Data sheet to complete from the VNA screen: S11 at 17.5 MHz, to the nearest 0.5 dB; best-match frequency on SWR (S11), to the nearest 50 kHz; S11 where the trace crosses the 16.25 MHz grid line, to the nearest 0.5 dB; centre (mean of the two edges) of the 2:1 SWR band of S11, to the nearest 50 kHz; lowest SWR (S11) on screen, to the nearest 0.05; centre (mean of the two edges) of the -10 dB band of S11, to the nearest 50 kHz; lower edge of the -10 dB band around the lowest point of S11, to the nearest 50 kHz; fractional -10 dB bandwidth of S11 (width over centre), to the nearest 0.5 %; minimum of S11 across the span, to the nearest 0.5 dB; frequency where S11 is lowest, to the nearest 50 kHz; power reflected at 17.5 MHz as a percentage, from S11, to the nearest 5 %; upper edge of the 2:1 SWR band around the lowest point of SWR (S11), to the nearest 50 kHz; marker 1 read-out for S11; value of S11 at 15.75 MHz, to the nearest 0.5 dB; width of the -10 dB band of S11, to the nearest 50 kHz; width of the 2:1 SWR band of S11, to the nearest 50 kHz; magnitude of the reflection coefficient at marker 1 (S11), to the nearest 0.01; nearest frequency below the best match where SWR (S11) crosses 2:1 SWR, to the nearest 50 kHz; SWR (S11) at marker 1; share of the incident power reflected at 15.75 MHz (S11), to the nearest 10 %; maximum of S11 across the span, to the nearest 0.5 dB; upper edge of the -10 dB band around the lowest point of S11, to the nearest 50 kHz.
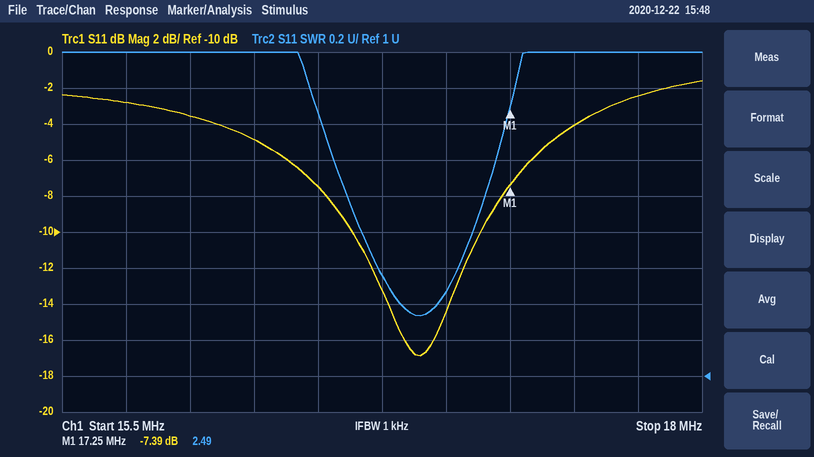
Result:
-4.0 dB
16.90 MHz
-5.0 dB
16.90 MHz
1.35
16.90 MHz
16.65 MHz
3.0 %
-17.0 dB
16.90 MHz
40 %
17.15 MHz
-7.39 dB
-3.0 dB
500 kHz
550 kHz
0.43
16.60 MHz
2.49
50 %
-1.5 dB
17.15 MHz
